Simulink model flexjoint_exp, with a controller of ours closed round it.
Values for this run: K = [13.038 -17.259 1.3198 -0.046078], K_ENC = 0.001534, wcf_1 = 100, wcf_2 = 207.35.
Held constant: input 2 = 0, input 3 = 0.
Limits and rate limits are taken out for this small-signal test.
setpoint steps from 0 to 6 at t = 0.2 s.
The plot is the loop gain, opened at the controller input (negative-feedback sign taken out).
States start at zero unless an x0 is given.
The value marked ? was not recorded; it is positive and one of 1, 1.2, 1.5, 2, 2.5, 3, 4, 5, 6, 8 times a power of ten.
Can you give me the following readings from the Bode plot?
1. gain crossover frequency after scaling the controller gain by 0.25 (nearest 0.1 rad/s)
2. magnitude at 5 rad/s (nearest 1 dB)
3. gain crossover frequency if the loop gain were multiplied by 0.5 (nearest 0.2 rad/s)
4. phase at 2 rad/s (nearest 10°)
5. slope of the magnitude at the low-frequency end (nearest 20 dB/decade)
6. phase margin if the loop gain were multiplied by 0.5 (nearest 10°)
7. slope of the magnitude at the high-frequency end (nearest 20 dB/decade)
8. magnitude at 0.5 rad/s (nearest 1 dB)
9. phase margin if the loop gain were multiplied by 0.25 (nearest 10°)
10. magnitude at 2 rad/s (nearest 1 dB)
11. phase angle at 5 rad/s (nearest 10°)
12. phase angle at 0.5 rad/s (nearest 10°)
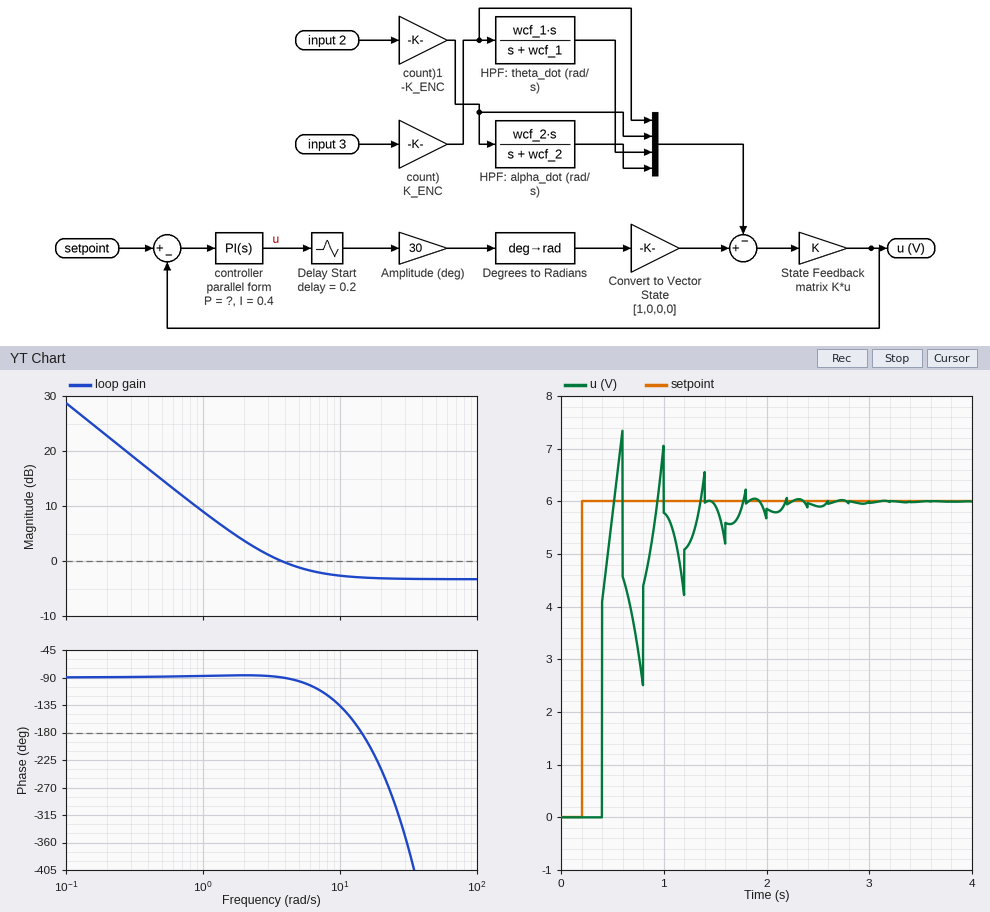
0.7 rad/s
-1 dB
1.4 rad/s
-90°
-20 dB/decade
90°
0 dB/decade
15 dB
90°
4 dB
-100°
-90°
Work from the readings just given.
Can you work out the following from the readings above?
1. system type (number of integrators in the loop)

1
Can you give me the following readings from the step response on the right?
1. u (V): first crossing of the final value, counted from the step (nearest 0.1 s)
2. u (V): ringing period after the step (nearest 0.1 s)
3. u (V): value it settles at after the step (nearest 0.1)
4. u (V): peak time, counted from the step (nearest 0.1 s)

0.3 s
0.4 s
6.0
0.4 s
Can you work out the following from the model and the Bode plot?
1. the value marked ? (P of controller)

0.1
